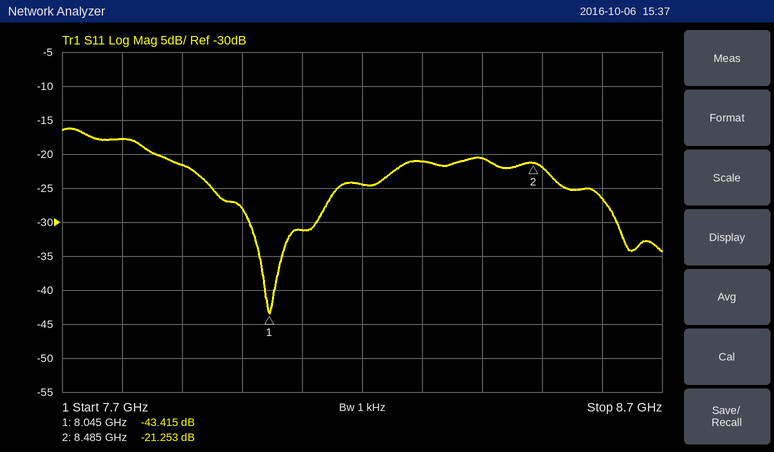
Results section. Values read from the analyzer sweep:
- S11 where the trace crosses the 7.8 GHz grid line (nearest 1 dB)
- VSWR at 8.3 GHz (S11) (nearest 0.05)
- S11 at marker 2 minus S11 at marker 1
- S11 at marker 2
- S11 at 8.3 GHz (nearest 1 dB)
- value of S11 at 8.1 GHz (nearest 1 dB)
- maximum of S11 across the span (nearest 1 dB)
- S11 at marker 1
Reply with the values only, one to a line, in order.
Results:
-18 dB
1.20
22.162 dB
-21.253 dB
-21 dB
-31 dB
-16 dB
-43.415 dB
